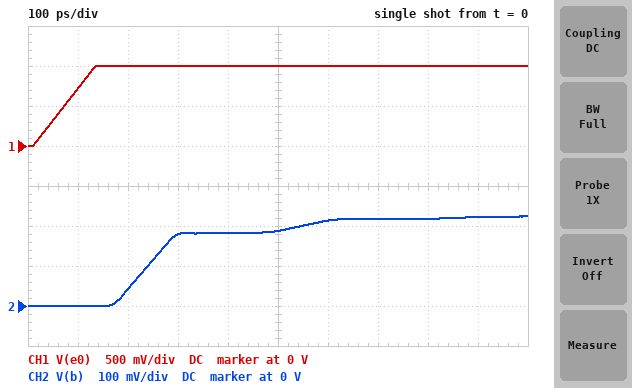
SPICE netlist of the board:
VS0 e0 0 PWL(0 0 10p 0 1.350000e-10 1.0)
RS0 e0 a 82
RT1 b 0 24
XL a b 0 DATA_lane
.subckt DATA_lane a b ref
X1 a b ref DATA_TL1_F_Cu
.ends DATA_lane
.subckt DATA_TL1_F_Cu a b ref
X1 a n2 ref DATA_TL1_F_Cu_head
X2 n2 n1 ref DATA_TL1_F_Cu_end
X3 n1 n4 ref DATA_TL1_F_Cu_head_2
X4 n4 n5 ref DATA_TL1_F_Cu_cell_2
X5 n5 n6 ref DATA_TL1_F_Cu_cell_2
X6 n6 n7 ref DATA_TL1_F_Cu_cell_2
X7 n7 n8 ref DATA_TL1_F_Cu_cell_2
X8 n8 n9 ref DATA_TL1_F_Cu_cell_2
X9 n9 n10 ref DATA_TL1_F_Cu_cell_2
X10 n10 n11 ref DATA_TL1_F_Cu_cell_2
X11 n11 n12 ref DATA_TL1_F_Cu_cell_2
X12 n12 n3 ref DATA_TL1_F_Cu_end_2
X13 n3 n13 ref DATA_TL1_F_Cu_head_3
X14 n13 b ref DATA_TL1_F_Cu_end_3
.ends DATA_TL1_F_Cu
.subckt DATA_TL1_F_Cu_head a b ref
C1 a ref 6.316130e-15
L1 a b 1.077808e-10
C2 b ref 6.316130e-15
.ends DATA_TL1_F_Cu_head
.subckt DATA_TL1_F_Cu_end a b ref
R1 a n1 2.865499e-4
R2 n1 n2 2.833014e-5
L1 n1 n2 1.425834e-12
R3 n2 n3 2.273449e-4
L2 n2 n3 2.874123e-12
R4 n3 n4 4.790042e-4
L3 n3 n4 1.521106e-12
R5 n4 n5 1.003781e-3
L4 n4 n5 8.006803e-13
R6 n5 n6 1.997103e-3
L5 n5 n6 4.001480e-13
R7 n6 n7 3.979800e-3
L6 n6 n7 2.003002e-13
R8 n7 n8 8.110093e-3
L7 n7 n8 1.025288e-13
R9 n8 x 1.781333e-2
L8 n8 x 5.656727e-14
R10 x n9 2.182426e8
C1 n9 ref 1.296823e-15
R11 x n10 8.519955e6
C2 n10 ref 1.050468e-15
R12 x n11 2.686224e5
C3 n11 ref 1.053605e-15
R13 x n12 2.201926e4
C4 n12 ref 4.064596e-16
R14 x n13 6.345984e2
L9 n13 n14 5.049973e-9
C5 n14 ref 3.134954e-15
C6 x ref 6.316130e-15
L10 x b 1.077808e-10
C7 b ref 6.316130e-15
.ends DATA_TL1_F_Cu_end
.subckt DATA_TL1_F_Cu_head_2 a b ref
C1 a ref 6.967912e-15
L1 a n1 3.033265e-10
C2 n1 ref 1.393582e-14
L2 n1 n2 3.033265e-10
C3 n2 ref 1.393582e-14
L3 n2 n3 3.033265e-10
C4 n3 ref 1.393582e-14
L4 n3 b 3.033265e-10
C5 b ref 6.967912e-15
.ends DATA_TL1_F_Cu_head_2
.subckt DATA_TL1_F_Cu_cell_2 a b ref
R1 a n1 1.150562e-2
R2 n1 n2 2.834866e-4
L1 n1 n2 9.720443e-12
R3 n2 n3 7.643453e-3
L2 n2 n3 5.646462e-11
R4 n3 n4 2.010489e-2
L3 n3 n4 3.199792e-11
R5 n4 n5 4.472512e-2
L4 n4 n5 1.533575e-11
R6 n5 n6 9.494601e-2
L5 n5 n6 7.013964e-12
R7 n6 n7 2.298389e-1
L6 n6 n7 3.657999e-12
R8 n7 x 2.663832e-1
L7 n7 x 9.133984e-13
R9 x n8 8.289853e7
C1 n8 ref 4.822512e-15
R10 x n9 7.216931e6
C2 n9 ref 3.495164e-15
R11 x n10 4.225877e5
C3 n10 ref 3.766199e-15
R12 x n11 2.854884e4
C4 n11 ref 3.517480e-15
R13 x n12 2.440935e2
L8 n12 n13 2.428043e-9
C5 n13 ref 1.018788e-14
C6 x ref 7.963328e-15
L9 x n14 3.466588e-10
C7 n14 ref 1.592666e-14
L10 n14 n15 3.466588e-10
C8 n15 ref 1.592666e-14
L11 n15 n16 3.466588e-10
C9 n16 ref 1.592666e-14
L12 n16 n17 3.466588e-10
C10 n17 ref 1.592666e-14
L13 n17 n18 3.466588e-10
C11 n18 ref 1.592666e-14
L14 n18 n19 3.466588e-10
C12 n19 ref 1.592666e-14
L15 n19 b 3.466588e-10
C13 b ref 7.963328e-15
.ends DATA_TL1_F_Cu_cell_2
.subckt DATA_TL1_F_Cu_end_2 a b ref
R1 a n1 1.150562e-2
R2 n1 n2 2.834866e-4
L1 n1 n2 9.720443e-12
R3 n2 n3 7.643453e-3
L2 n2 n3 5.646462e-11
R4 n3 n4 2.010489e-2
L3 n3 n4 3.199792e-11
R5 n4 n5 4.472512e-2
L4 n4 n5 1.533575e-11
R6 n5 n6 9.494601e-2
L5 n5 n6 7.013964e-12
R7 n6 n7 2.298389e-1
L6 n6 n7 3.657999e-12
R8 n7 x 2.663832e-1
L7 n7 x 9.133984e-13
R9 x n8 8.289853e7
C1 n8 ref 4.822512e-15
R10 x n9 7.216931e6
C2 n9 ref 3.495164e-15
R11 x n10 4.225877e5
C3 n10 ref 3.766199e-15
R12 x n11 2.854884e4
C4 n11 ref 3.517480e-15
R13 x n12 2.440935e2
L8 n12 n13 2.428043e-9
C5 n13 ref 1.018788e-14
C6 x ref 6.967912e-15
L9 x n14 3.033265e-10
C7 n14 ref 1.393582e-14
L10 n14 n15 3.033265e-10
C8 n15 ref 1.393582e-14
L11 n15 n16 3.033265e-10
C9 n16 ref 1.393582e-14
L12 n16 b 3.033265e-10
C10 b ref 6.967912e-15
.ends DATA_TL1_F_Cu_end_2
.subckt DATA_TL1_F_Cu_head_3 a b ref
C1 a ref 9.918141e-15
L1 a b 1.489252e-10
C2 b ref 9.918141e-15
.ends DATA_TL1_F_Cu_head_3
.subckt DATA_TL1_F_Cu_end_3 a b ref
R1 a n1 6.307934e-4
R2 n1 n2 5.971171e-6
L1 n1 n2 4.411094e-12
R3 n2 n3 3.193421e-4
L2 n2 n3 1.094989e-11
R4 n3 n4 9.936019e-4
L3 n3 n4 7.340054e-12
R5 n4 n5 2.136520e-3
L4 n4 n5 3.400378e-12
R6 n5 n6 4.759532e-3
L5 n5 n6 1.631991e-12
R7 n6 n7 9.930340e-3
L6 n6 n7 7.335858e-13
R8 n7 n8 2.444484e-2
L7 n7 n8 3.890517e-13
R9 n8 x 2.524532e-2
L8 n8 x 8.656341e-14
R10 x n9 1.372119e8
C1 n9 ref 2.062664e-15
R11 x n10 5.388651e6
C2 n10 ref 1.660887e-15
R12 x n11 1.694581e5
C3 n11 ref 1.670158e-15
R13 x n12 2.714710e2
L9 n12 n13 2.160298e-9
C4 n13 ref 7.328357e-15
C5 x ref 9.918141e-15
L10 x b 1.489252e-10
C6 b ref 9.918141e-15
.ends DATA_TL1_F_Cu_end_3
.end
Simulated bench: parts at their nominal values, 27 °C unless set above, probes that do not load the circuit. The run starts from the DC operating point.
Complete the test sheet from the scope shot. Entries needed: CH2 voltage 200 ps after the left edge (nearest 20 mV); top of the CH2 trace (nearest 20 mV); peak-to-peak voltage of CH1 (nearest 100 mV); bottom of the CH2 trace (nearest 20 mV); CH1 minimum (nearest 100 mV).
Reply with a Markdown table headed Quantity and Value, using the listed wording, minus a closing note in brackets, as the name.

| Quantity | Value |
|---|---|
| CH2 voltage 200 ps after the left edge | 40 mV |
| top of the CH2 trace | 220 mV |
| peak-to-peak voltage of CH1 | 1.0 V |
| bottom of the CH2 trace | 0 V |
| CH1 minimum | 0 V |
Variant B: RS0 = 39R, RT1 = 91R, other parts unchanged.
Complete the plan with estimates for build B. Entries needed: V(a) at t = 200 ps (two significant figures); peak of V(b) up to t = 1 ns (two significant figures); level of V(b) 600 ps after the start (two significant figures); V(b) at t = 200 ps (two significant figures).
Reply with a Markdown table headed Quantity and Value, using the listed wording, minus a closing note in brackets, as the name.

| Quantity | Value |
|---|---|
| V(a) at t = 200 ps | 780 mV |
| peak of V(b) up to t = 1 ns | 700 mV |
| level of V(b) 600 ps after the start | 680 mV |
| V(b) at t = 200 ps | 140 mV |
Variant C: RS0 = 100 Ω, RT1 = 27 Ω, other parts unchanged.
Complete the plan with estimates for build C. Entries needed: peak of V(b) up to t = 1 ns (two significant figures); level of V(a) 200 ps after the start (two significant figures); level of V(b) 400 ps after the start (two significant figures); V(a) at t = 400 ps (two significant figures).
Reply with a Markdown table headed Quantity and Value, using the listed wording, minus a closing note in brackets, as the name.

| Quantity | Value |
|---|---|
| peak of V(b) up to t = 1 ns | 210 mV |
| level of V(a) 200 ps after the start | 580 mV |
| level of V(b) 400 ps after the start | 190 mV |
| V(a) at t = 400 ps | 400 mV |
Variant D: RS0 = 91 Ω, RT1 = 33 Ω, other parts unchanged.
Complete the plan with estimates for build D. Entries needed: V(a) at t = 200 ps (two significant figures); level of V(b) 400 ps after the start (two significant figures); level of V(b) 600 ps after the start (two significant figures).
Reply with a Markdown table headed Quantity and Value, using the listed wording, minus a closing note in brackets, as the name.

| Quantity | Value |
|---|---|
| V(a) at t = 200 ps | 610 mV |
| level of V(b) 400 ps after the start | 230 mV |
| level of V(b) 600 ps after the start | 260 mV |
